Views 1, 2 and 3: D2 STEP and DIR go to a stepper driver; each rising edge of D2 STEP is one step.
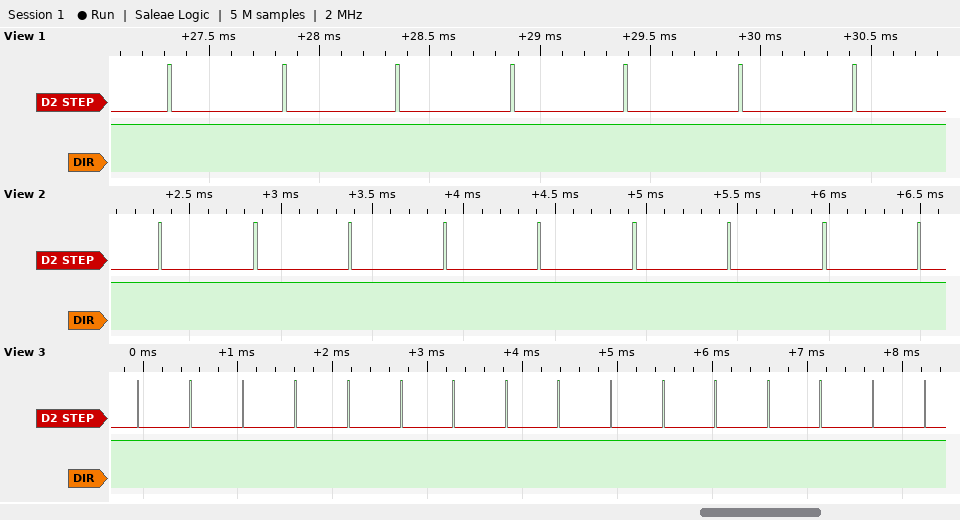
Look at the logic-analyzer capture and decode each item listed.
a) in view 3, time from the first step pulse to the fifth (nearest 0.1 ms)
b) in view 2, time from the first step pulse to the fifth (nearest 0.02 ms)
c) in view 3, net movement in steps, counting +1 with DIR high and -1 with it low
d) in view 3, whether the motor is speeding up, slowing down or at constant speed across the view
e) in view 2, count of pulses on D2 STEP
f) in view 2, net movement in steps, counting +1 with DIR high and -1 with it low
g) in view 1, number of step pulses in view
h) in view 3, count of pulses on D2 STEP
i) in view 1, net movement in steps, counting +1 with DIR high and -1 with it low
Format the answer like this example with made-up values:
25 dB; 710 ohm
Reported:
2.2 ms; 2.08 ms; +16; constant speed; 9; +9; 7; 16; +7
